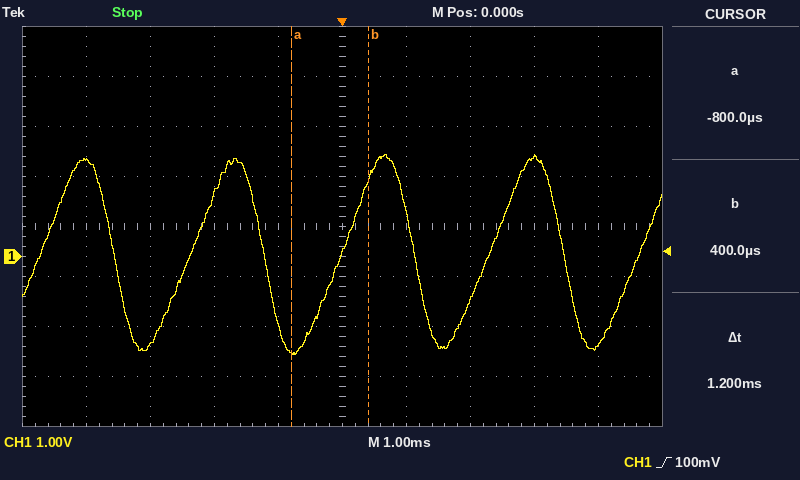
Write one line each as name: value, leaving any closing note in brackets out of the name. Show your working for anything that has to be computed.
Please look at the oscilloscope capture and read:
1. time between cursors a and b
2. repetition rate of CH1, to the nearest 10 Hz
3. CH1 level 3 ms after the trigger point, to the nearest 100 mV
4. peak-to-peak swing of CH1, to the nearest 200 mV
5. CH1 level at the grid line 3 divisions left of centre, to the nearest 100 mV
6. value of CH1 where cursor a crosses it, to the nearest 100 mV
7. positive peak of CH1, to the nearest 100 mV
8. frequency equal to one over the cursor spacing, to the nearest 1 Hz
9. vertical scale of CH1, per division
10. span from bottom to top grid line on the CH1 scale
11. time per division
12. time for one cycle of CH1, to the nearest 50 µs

time between cursors a and b: 1.2 ms
repetition rate of CH1, to the nearest 10 Hz: 1 / 2.35 ms ≈ 426 Hz, so 430 Hz to the nearest 10 Hz
CH1 level 3 ms after the trigger point, to the nearest 100 mV: 2.0 V
peak-to-peak swing of CH1, to the nearest 200 mV: 4.0 V
CH1 level at the grid line 3 divisions left of centre, to the nearest 100 mV: -1.8 V
value of CH1 where cursor a crosses it, to the nearest 100 mV: -1.9 V
positive peak of CH1, to the nearest 100 mV: 2.0 V
frequency equal to one over the cursor spacing, to the nearest 1 Hz: 1 / 1.2 ms ≈ 833 Hz
vertical scale of CH1, per division: 1 V
span from bottom to top grid line on the CH1 scale: 8 V
time per division: 1 ms
time for one cycle of CH1, to the nearest 50 µs: 2.35 ms
